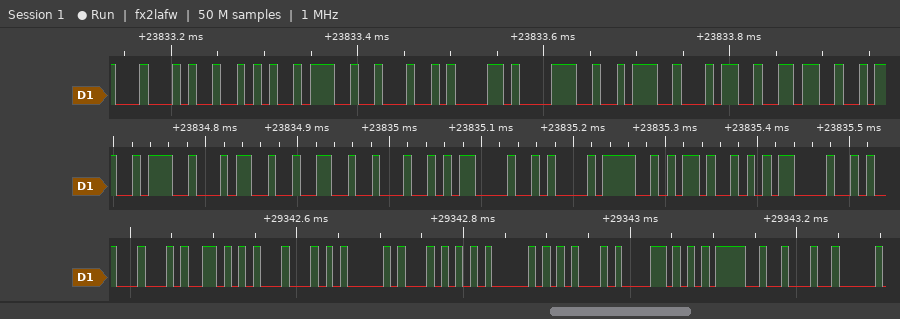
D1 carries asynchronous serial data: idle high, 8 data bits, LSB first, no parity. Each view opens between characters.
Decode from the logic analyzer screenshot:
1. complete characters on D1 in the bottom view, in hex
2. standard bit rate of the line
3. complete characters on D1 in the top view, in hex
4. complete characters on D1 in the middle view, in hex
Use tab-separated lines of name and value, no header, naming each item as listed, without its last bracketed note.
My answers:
complete characters on D1 in the bottom view, in hex	44, 56, 44, 41, 54, 41, 45, 58, 3D, 22
standard bit rate of the line	115200 baud
complete characters on D1 in the top view, in hex	44, 52, 3A, 22, 61, 38, 3A, 34, 36
complete characters on D1 in the middle view, in hex	3A, 34, 32, 22, 0D, 0A, 4F, 4B, 0D
